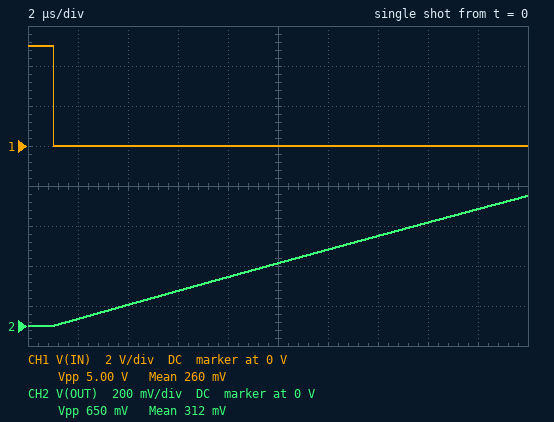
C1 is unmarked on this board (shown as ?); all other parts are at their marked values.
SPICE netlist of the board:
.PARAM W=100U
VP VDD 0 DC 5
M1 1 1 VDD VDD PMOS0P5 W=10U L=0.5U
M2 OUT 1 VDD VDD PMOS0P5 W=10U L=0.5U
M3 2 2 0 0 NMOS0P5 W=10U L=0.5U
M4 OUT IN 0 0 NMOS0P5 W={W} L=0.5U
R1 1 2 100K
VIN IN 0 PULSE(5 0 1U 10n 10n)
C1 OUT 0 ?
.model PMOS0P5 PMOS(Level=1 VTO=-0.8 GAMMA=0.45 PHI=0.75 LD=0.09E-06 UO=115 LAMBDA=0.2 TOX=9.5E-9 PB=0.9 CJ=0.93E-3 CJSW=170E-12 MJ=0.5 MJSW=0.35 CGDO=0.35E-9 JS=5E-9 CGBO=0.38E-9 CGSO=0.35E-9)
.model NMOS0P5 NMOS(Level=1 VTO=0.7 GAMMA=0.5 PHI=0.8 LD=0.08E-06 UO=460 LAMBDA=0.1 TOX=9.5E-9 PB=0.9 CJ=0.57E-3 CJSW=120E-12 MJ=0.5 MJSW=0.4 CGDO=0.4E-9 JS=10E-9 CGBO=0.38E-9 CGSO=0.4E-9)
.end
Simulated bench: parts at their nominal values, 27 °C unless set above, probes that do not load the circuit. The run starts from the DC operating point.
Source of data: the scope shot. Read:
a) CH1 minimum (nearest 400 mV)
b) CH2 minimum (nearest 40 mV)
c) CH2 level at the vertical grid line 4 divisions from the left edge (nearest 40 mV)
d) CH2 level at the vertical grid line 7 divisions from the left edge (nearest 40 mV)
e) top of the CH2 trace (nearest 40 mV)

0 V
0 V
240 mV
440 mV
640 mV
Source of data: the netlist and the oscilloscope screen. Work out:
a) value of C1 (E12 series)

1.5 nF
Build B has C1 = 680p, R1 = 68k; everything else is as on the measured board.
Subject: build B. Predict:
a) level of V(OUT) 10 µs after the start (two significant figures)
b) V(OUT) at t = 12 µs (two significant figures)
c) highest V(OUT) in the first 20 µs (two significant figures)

960 mV
1.2 V
1.9 V
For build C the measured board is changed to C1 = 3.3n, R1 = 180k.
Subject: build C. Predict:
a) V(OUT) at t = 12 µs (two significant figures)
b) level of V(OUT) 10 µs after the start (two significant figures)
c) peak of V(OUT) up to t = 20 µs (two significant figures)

100 mV
83 mV
170 mV
